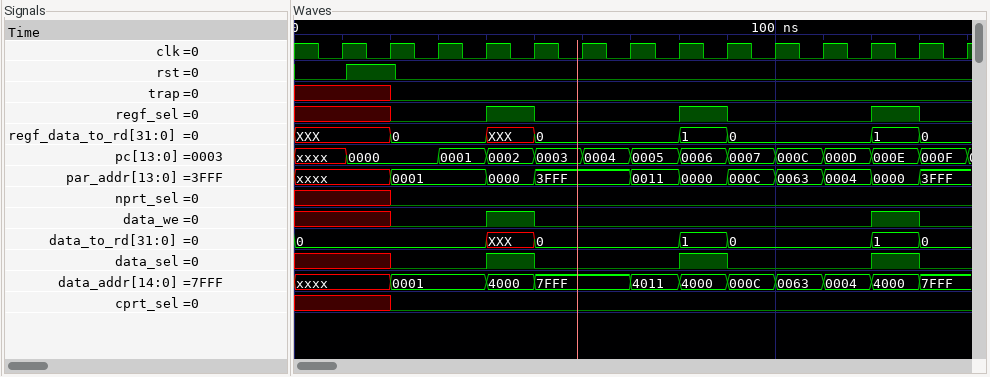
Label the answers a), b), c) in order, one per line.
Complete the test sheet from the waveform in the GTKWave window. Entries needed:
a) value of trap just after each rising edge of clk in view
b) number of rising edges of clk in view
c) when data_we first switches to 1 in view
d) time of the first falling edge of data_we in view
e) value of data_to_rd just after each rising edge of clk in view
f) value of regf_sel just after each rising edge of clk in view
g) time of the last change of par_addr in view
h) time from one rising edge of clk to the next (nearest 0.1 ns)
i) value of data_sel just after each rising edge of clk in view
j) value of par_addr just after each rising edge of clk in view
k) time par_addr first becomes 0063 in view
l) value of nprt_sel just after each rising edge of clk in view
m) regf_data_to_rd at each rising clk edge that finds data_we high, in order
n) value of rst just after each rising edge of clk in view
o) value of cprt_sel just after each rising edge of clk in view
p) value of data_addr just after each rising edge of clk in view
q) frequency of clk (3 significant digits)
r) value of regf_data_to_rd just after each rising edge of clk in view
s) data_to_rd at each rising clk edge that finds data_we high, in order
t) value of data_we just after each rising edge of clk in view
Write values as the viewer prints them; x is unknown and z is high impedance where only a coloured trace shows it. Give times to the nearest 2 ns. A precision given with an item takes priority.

a) x 0 0 0 0 0 0 0 0 0 0 0 0 0
b) 14
c) 40 ns
d) 50 ns
e) 0, 0, 0, XXX, 0, 0, 0, 1, 0, 0, 0, 1, 0, 0
f) x 0 0 1 0 0 0 1 0 0 0 1 0 0
g) 130 ns
h) 10 ns
i) x 0 0 1 0 0 0 1 0 0 0 1 0 0
j) xxxx, 0001, 0001, 0000, 3FFF, 3FFF, 0011, 0000, 000C, 0063, 0004, 0000, 3FFF, 3FFF
k) 100 ns
l) x 0 0 0 0 0 0 0 0 0 0 0 0 0
m) XXX, 1
n) 0 1 0 0 0 0 0 0 0 0 0 0 0 0
o) x 0 0 0 0 0 0 0 0 0 0 0 0 0
p) xxxx, 0001, 0001, 4000, 7FFF, 7FFF, 4011, 4000, 000C, 0063, 0004, 4000, 7FFF, 7FFF
q) 100 MHz
r) XXX, 0, 0, XXX, 0, 0, 0, 1, 0, 0, 0, 1, 0, 0
s) XXX, 1
t) x 0 0 1 0 0 0 0 0 0 0 1 0 0
